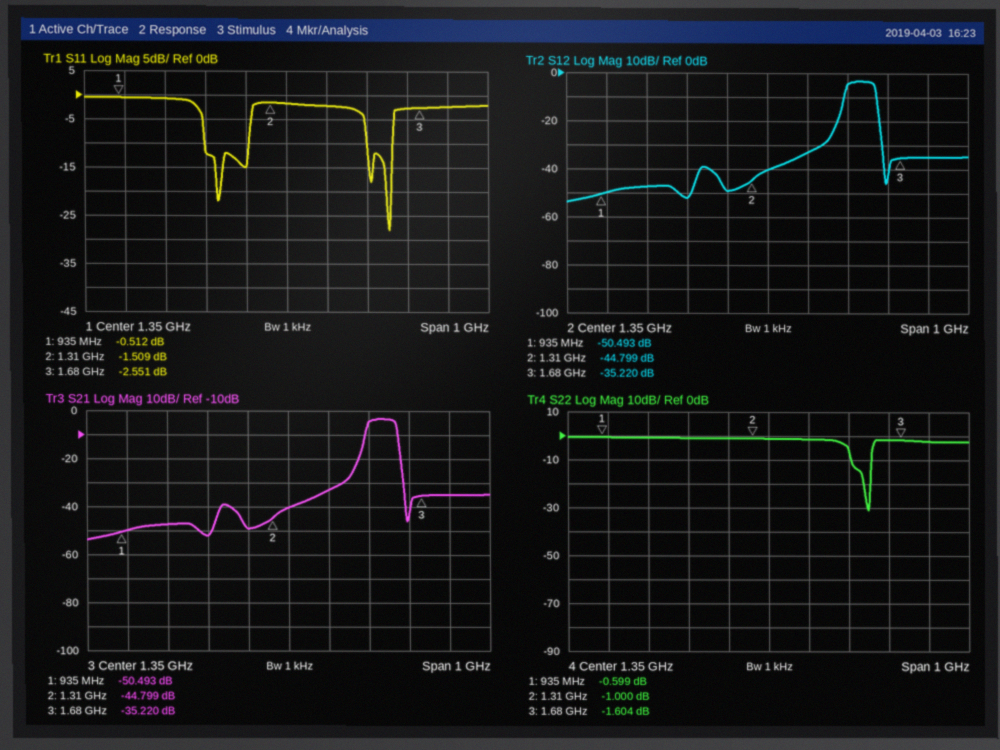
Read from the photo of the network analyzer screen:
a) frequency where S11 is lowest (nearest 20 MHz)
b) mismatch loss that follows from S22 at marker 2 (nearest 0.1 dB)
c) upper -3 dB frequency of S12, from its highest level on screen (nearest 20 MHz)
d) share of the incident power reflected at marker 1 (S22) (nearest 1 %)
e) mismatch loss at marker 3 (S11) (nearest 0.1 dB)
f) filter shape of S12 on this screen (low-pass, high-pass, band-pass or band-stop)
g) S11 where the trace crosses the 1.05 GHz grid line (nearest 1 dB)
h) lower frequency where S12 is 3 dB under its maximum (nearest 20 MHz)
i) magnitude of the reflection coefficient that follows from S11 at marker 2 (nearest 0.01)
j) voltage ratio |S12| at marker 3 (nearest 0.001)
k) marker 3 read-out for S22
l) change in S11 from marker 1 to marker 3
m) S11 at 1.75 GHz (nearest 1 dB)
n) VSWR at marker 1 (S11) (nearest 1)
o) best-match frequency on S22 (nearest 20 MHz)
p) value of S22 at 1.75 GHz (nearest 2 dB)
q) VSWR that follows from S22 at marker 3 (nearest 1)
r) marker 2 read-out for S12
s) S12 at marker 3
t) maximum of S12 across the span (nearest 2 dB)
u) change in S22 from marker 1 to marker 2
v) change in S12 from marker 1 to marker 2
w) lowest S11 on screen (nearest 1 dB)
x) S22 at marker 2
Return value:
1.60 GHz
6.9 dB
1.62 GHz
87 %
3.5 dB
band-pass
-1 dB
1.54 GHz
0.84
0.017
-1.604 dB
-2.039 dB
-2 dB
34
1.60 GHz
-2 dB
11
-44.799 dB
-35.220 dB
-4 dB
-0.401 dB
5.694 dB
-28 dB
-1.000 dB
